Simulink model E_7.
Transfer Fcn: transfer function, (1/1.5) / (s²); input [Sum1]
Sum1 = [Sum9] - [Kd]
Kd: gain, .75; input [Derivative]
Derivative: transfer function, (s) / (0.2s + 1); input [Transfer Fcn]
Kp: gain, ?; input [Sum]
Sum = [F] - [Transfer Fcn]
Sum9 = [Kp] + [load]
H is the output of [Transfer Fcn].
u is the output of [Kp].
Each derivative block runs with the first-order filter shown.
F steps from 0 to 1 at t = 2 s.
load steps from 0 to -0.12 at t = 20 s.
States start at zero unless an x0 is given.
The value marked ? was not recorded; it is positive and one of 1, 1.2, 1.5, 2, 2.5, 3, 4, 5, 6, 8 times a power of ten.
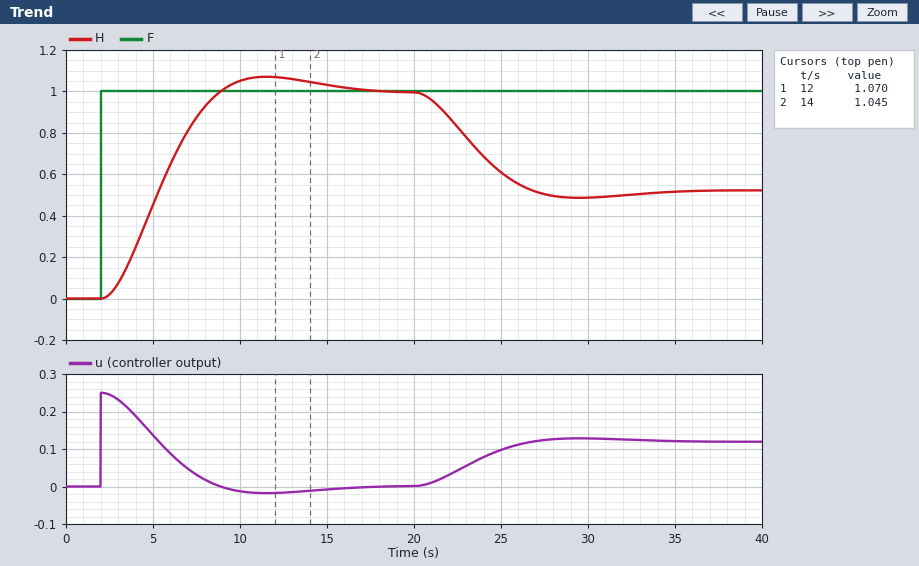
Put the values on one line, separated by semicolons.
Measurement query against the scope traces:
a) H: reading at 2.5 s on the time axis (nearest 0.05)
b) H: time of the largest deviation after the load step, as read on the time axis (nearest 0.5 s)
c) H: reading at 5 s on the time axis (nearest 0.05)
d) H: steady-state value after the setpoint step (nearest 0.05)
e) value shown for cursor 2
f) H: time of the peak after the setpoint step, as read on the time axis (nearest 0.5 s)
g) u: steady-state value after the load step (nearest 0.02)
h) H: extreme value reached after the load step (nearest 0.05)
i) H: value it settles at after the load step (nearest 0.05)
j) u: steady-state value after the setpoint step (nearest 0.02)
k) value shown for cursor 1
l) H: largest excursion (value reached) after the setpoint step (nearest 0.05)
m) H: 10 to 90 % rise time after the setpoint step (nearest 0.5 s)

0.00; 29.5 s; 0.45; 1.00; 1.045; 11.5 s; 0.12; 0.50; 0.50; 0.00; 1.070; 1.05; 4.5 s
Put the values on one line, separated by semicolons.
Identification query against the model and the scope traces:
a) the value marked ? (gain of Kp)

0.25
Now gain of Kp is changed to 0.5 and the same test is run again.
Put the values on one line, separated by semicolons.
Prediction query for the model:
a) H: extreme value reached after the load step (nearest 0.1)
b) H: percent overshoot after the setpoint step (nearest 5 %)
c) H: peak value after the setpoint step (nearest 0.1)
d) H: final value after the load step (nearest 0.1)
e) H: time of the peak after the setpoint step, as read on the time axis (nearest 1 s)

0.7; 20 %; 1.2; 0.8; 8 s
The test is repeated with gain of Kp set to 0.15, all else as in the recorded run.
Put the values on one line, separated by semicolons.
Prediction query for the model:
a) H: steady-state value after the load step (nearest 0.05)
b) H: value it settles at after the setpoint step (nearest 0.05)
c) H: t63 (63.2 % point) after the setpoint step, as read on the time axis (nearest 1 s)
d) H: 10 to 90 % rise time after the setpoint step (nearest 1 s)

0.20; 1.00; 8 s; 8 s
